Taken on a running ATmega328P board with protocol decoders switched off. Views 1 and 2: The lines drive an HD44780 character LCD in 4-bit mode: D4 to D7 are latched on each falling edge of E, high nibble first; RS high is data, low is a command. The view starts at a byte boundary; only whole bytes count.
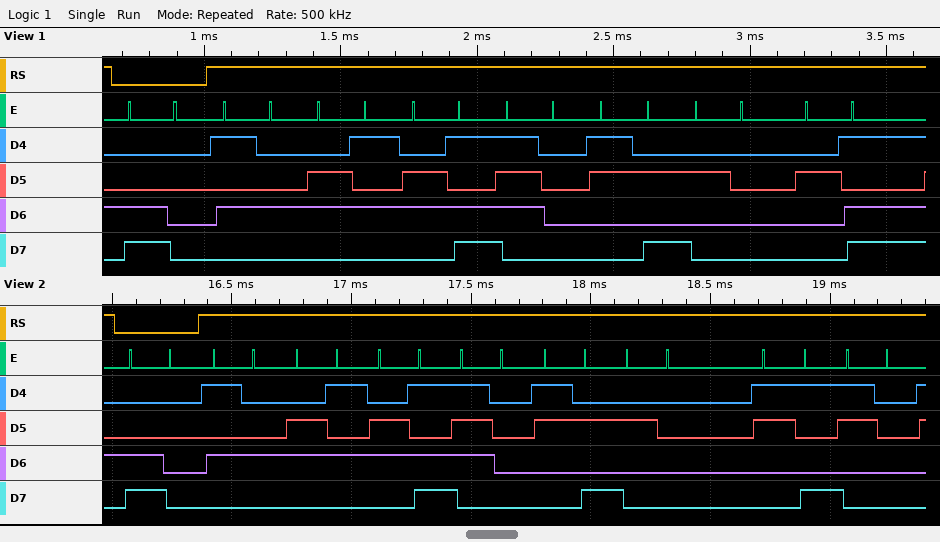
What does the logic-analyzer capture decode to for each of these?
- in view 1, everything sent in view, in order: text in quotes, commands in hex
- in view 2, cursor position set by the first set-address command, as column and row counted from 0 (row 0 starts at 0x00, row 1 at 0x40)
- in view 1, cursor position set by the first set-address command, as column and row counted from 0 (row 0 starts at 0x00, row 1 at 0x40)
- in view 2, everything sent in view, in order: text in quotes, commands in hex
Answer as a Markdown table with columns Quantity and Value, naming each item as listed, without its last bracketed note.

| Quantity | Value |
|---|---|
| in view 1, everything sent in view, in order: text in quotes, commands in hex | 0xC0 "Temp: -" |
| in view 2, cursor position set by the first set-address command, as column and row counted from 0 | column 0, row 1 |
| in view 1, cursor position set by the first set-address command, as column and row counted from 0 | column 0, row 1 |
| in view 2, everything sent in view, in order: text in quotes, commands in hex | 0xC0 "Temp: 90" |
